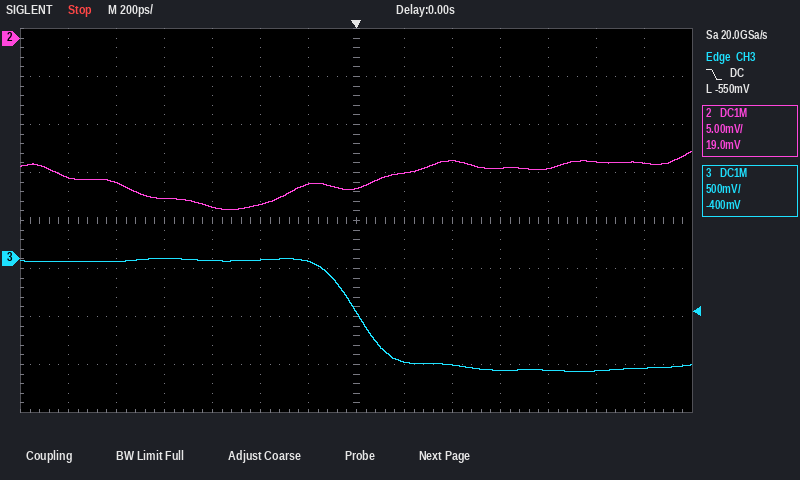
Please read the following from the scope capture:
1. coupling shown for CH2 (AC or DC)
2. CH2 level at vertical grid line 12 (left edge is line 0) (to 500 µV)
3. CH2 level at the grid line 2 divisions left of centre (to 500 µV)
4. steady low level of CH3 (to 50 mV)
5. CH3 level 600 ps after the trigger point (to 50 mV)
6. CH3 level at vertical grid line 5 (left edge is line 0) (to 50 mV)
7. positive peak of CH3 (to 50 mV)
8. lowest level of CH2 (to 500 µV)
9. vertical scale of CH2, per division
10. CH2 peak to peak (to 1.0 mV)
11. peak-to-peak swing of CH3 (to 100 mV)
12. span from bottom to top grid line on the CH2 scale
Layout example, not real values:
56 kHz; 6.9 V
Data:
DC; -13.0 mV; -17.5 mV; -1.15 V; -1.15 V; 0 mV; 0 mV; -18.0 mV; 5 mV; 6.0 mV; 1.20 V; 40 mV
